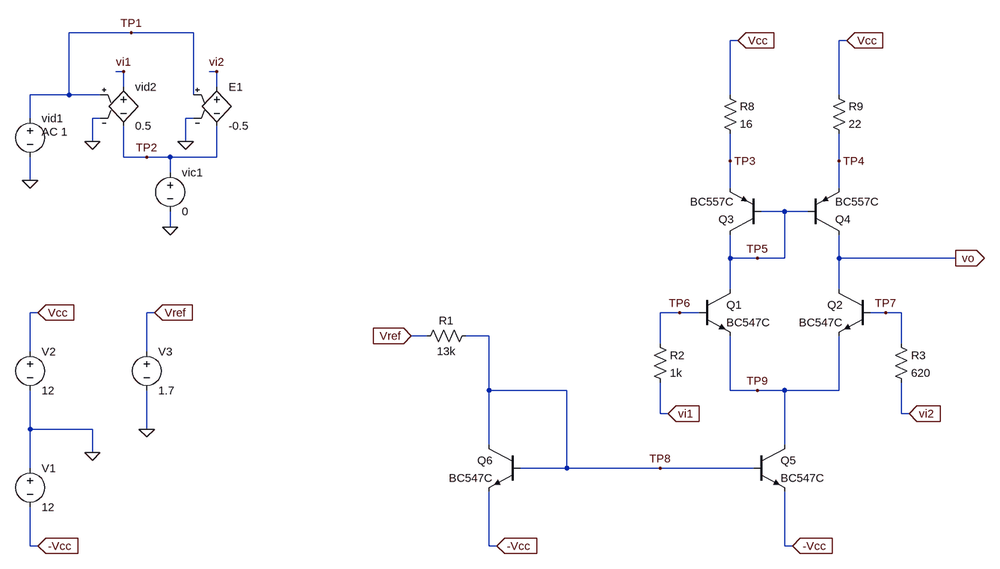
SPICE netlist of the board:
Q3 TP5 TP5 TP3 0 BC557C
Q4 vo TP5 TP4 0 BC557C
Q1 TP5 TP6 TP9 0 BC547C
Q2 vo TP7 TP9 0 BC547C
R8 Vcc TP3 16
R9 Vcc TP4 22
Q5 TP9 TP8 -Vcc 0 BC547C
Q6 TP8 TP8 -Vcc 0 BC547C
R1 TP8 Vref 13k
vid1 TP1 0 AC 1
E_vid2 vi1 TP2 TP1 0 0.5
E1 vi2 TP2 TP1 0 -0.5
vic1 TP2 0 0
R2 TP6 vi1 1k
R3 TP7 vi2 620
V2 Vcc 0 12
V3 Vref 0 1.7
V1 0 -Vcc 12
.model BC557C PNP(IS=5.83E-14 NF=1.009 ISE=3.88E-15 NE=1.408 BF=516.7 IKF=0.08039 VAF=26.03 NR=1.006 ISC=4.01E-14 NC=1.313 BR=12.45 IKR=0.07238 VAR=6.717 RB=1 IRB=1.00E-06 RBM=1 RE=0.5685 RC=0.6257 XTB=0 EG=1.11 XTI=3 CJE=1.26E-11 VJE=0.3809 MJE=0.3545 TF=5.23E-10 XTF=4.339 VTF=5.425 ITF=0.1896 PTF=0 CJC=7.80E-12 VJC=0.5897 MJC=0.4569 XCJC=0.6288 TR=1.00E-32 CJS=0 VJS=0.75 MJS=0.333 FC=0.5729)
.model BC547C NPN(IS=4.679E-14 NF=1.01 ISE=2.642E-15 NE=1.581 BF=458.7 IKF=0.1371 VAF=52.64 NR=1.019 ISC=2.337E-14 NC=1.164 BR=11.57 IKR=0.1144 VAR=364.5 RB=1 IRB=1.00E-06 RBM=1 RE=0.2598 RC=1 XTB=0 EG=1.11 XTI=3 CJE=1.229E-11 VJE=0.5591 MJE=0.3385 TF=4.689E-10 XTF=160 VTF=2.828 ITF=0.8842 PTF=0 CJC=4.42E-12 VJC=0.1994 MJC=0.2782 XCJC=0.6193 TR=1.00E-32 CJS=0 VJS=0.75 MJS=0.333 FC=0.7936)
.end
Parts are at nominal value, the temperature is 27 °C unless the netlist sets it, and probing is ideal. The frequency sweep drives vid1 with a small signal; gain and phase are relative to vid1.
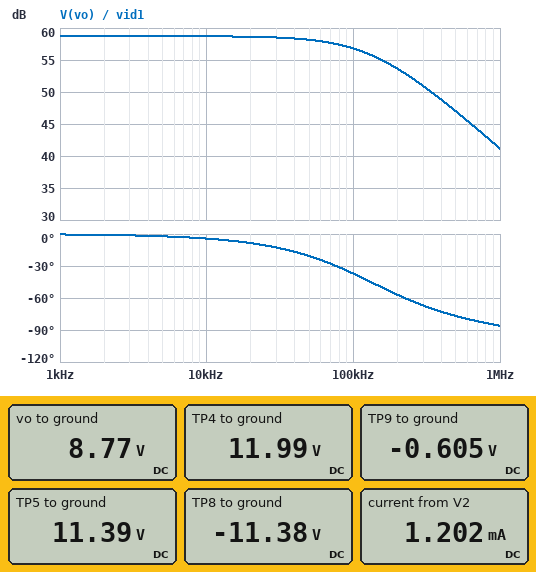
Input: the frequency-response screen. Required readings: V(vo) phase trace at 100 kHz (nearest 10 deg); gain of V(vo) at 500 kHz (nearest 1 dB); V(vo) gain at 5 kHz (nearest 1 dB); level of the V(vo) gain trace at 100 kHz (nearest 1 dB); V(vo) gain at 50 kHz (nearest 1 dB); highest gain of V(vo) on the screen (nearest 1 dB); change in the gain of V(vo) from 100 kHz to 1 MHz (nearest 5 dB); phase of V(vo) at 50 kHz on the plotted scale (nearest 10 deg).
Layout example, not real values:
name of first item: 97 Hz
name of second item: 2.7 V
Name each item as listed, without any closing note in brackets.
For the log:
V(vo) phase trace at 100 kHz: -40 deg
gain of V(vo) at 500 kHz: 47 dB
V(vo) gain at 5 kHz: 59 dB
level of the V(vo) gain trace at 100 kHz: 57 dB
V(vo) gain at 50 kHz: 58 dB
highest gain of V(vo) on the screen: 59 dB
change in the gain of V(vo) from 100 kHz to 1 MHz: -15 dB
phase of V(vo) at 50 kHz on the plotted scale: -20 deg
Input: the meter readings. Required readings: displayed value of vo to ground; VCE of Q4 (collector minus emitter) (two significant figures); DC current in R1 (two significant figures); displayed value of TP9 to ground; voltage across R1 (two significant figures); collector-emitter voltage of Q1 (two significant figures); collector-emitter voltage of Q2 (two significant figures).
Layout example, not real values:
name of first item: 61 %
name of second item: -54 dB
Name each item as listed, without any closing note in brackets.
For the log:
displayed value of vo to ground: 8.77 V
VCE of Q4 (collector minus emitter): -3.2 V
DC current in R1: 1.0 mA
displayed value of TP9 to ground: -0.605 V
voltage across R1: 13 V
collector-emitter voltage of Q1: 12 V
collector-emitter voltage of Q2: 9.4 V
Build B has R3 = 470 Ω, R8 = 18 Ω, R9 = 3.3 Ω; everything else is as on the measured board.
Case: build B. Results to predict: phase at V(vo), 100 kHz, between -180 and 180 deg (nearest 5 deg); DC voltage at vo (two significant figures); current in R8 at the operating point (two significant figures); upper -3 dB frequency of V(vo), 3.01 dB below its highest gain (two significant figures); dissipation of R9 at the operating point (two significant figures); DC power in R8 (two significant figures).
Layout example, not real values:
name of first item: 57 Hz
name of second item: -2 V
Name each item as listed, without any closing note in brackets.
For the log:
phase at V(vo), 100 kHz, between -180 and 180 deg: 0 deg
DC voltage at vo: 12 V
current in R8 at the operating point: 580 µA
upper -3 dB frequency of V(vo), 3.01 dB below its highest gain: 4.3 MHz
dissipation of R9 at the operating point: 1.3 µW
DC power in R8: 6.0 µW
